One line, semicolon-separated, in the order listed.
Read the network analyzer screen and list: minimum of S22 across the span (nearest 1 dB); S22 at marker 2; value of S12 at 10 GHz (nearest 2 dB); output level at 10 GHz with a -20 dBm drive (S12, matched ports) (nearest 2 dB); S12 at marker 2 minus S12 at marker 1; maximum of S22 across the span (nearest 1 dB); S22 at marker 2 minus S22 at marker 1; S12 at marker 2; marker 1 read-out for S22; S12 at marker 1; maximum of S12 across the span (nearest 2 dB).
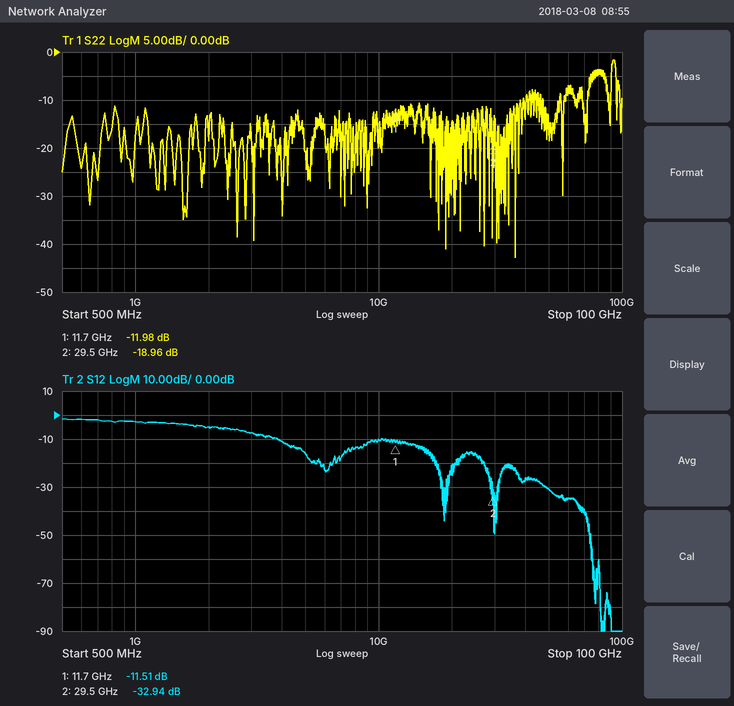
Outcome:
-43 dB; -18.96 dB; -10 dB; -30 dBm; -21.43 dB; -2 dB; -6.98 dB; -32.94 dB; -11.98 dB; -11.51 dB; -2 dB
